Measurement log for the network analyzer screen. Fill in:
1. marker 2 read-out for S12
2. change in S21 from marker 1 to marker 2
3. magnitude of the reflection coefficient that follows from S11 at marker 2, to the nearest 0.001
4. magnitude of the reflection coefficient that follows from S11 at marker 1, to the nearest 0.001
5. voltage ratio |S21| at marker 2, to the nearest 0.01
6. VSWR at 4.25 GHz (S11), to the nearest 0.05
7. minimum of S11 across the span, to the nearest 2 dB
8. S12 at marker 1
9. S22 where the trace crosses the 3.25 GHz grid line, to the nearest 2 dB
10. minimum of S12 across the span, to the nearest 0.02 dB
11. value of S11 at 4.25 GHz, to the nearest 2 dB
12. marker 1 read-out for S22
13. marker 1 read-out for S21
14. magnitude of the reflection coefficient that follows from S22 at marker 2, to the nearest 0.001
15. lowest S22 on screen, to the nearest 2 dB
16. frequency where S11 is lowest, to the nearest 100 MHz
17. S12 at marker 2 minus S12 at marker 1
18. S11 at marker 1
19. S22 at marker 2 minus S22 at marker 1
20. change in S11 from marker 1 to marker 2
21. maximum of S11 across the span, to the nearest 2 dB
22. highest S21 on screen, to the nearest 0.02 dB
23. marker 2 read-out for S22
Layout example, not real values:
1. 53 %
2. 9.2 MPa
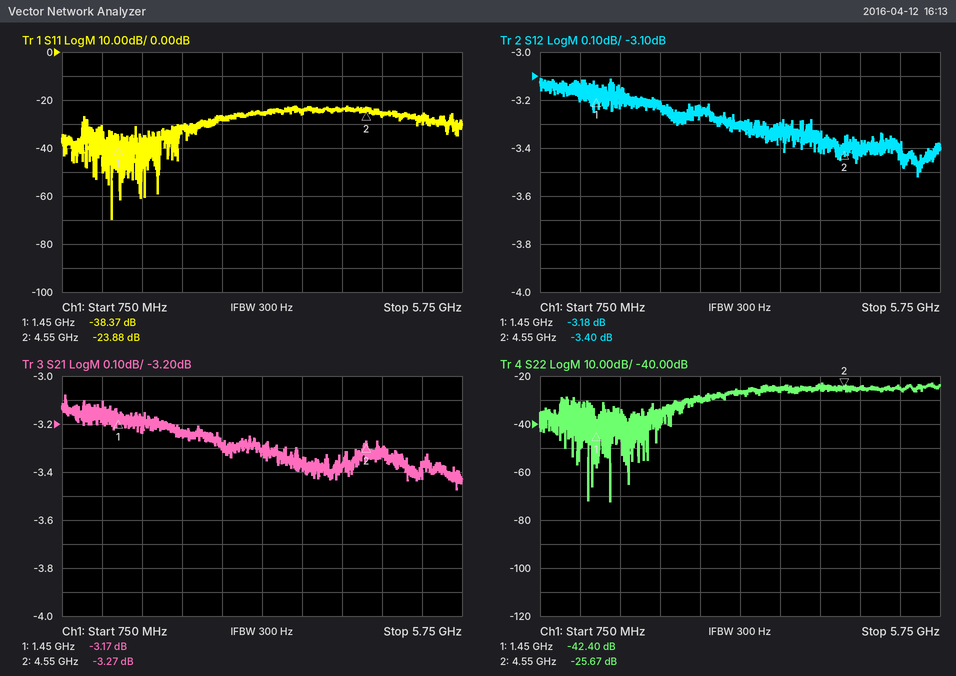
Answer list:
1. -3.40 dB
2. -0.10 dB
3. 0.064
4. 0.012
5. 0.69
6. 1.15
7. -70 dB
8. -3.18 dB
9. -26 dB
10. -3.52 dB
11. -24 dB
12. -42.40 dB
13. -3.17 dB
14. 0.052
15. -72 dB
16. 1.4 GHz
17. -0.22 dB
18. -38.37 dB
19. 16.73 dB
20. 14.49 dB
21. -22 dB
22. -3.08 dB
23. -25.67 dB
